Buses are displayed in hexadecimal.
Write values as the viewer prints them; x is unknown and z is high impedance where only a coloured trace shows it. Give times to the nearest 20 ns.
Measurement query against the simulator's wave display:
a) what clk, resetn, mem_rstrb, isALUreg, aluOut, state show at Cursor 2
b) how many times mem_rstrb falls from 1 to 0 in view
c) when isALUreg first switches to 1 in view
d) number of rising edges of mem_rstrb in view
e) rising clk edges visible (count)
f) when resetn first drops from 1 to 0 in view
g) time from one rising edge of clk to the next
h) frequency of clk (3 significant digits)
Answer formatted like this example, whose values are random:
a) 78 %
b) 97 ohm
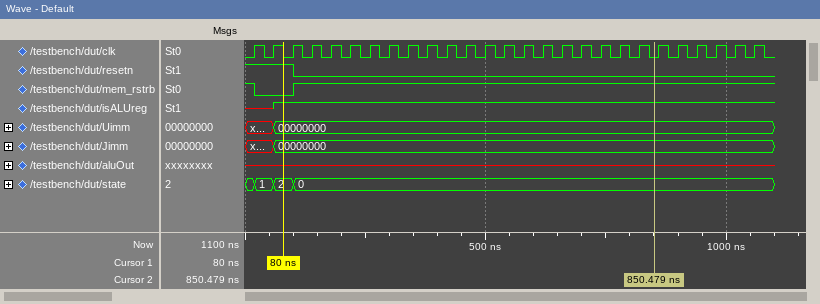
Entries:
a) clk=0, resetn=0, mem_rstrb=1, isALUreg=1, aluOut=x, state=0
b) 1
c) 60 ns
d) 1
e) 27
f) 100 ns
g) 40 ns
h) 25.0 MHz
